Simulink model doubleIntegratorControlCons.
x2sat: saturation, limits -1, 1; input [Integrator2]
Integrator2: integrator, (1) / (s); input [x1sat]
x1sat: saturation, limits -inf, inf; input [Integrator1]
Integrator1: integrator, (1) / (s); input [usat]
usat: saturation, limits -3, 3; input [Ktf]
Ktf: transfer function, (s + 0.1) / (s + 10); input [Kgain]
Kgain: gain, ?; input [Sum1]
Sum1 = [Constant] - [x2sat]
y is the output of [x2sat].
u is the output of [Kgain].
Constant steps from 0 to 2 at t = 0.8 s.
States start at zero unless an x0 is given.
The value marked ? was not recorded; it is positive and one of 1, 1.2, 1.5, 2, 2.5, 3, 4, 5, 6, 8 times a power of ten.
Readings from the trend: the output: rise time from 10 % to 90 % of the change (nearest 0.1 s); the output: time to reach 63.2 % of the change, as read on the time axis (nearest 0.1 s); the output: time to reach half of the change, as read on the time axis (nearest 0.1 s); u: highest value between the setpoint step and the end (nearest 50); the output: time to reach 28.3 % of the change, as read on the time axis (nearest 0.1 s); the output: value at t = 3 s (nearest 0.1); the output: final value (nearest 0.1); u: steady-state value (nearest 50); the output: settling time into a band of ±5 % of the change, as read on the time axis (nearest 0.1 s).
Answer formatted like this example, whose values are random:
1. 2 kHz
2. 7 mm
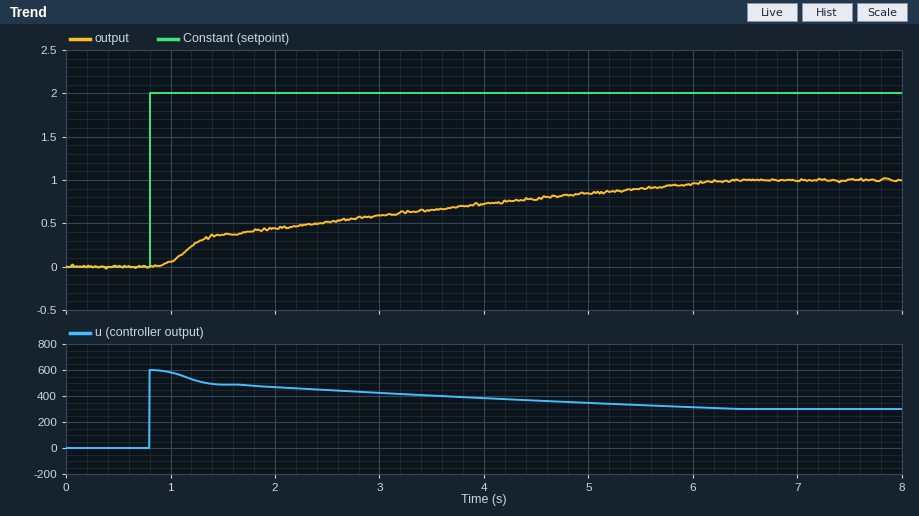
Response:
1. 4.4 s
2. 3.3 s
3. 2.4 s
4. 600
5. 1.3 s
6. 0.6
7. 1.0
8. 300
9. 6.0 s
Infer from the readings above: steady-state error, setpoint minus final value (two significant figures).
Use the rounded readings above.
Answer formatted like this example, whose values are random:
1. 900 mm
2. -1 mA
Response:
1. 1.0
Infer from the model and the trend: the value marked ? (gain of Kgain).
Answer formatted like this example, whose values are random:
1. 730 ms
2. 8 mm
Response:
1. 300
